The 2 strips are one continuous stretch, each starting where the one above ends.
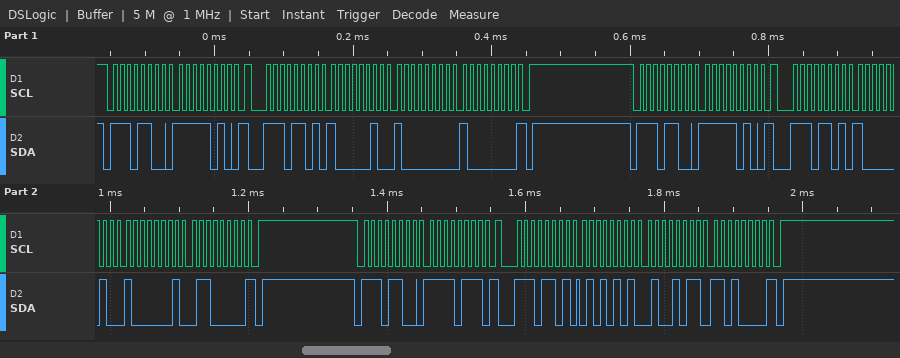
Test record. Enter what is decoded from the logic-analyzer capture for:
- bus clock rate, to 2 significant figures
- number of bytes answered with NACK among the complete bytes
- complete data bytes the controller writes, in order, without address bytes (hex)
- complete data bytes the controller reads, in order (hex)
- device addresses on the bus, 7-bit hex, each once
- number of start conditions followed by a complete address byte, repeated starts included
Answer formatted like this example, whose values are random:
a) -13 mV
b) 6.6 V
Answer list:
a) 100 kHz
b) 3
c) FA FA F7
d) 82 80 80 82 81 60 55 4B D0
e) 0x76
f) 6
